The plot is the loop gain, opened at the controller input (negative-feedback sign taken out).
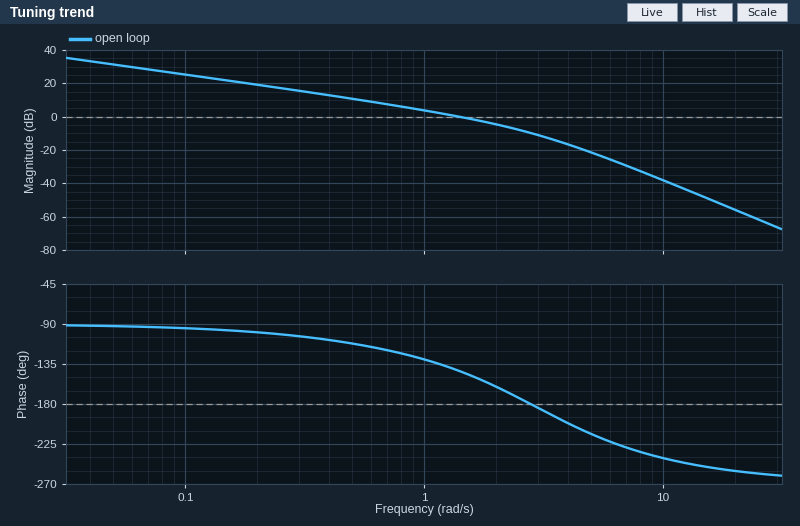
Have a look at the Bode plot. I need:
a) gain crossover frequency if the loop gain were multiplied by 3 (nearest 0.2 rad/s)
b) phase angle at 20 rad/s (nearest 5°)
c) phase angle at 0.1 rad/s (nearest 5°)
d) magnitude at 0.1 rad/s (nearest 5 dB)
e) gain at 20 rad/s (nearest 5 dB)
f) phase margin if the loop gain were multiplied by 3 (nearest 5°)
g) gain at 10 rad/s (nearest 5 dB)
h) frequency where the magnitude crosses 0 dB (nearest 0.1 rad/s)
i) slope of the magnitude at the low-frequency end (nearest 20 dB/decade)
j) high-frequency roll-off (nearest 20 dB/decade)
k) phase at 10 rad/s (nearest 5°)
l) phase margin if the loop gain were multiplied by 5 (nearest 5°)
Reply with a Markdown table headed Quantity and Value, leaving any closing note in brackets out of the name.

| Quantity | Value |
|---|---|
| gain crossover frequency if the loop gain were multiplied by 3 | 2.8 rad/s |
| phase angle at 20 rad/s | -255° |
| phase angle at 0.1 rad/s | -95° |
| magnitude at 0.1 rad/s | 25 dB |
| gain at 20 rad/s | -55 dB |
| phase margin if the loop gain were multiplied by 3 | 0° |
| gain at 10 rad/s | -40 dB |
| frequency where the magnitude crosses 0 dB | 1.4 rad/s |
| slope of the magnitude at the low-frequency end | -20 dB/decade |
| high-frequency roll-off | -60 dB/decade |
| phase at 10 rad/s | -240° |
| phase margin if the loop gain were multiplied by 5 | -15° |
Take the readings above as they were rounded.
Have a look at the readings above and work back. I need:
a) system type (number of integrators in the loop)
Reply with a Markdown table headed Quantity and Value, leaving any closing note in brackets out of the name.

| Quantity | Value |
|---|---|
| system type | 1 |
